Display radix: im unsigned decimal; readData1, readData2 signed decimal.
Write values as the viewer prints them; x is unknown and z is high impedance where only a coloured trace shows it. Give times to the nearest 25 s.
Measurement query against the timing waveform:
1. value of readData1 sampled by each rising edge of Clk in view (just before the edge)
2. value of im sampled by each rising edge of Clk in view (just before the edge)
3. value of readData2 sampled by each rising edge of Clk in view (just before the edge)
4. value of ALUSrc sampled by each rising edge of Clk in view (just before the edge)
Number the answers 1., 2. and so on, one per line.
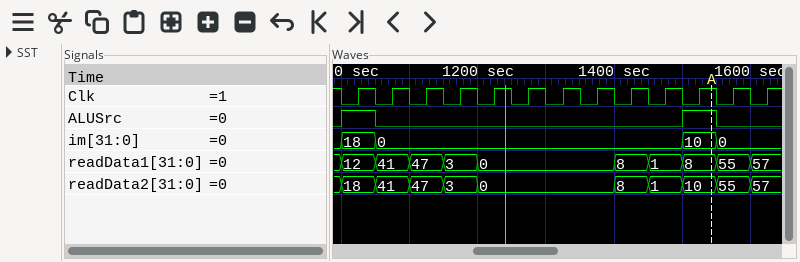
1. 12, 41, 47, 3, 0, 0, 0, 0, 8, 1, 8, 55, 57
2. 18, 0, 0, 0, 0, 0, 0, 0, 0, 0, 10, 0, 0
3. 18, 41, 47, 3, 0, 0, 0, 0, 8, 1, 10, 55, 57
4. 1 0 0 0 0 0 0 0 0 0 1 0 0
